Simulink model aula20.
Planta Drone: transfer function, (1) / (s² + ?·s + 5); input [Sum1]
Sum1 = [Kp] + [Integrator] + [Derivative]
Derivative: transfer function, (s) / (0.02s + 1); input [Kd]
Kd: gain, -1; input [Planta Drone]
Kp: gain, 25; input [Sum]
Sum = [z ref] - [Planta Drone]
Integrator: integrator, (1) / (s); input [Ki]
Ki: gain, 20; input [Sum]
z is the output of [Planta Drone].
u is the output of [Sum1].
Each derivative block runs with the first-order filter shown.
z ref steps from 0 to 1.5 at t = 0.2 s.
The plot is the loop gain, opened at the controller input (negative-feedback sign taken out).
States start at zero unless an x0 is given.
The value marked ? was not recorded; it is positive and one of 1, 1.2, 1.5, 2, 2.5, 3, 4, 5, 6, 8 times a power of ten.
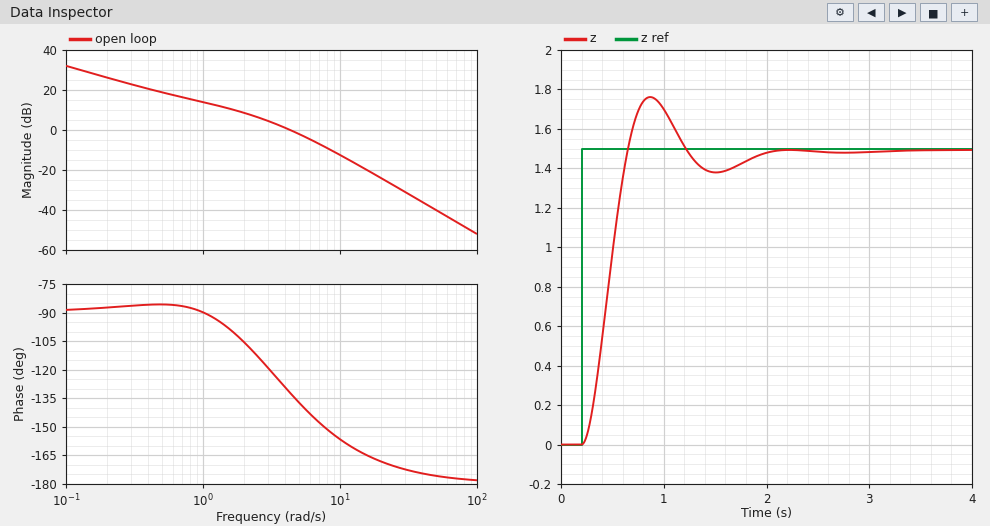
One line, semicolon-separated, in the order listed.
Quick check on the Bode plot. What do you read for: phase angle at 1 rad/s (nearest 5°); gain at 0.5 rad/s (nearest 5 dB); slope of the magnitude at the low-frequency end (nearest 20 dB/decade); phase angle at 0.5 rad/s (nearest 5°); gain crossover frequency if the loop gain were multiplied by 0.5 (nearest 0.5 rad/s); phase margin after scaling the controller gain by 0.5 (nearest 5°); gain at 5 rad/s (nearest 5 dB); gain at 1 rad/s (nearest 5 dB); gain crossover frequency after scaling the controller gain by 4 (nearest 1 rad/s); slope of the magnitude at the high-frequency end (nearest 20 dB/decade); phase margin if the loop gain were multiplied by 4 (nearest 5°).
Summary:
-90°; 20 dB; -20 dB/decade; -85°; 2.5 rad/s; 65°; 0 dB; 15 dB; 10 rad/s; -40 dB/decade; 25°
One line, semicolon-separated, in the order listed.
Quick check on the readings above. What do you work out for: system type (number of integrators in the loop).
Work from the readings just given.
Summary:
1
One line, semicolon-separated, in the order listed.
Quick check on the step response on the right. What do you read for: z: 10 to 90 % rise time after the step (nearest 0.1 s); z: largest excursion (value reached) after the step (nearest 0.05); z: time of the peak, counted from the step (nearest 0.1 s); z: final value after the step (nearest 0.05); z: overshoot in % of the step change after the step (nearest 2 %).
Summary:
0.3 s; 1.75; 0.7 s; 1.50; 18 %
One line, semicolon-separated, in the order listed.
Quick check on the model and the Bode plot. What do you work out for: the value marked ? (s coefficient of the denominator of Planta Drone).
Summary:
4
